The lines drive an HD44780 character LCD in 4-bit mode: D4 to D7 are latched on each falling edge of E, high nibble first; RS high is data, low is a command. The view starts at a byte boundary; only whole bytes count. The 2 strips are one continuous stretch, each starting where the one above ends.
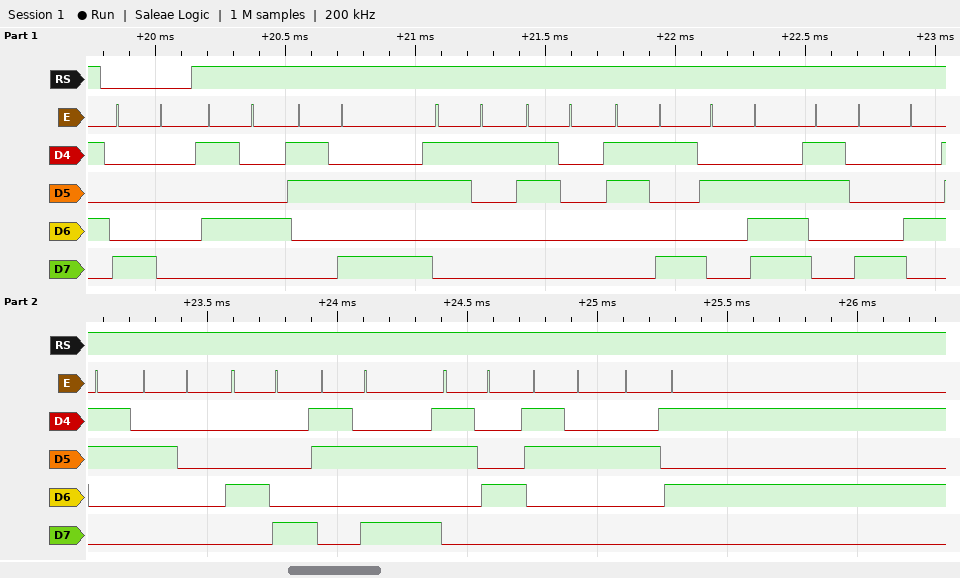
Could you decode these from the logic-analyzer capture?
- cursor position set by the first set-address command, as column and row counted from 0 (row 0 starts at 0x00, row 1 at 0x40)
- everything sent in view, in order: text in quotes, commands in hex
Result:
column 0, row 0
0x80 "T:109.8C H:42%"
